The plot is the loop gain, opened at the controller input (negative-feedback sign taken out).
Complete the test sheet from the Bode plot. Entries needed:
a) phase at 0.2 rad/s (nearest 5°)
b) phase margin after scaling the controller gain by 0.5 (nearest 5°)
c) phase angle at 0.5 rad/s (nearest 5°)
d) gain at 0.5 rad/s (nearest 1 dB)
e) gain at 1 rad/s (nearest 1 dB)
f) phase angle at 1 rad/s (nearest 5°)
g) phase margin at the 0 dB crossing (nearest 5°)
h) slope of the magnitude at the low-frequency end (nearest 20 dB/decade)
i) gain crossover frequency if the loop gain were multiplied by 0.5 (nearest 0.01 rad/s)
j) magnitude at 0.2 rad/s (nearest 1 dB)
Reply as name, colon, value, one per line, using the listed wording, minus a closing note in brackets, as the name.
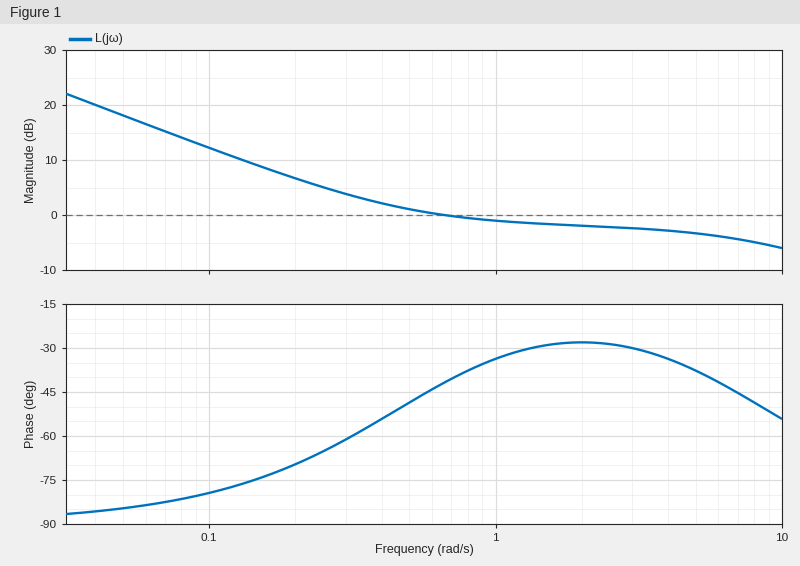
phase at 0.2 rad/s: -70°
phase margin after scaling the controller gain by 0.5: 110°
phase angle at 0.5 rad/s: -50°
gain at 0.5 rad/s: 1 dB
gain at 1 rad/s: -1 dB
phase angle at 1 rad/s: -35°
phase margin at the 0 dB crossing: 140°
slope of the magnitude at the low-frequency end: -20 dB/decade
gain crossover frequency if the loop gain were multiplied by 0.5: 0.22 rad/s
magnitude at 0.2 rad/s: 7 dB
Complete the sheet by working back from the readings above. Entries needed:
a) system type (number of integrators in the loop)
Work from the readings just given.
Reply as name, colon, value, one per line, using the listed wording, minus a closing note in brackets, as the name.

system type: 1
